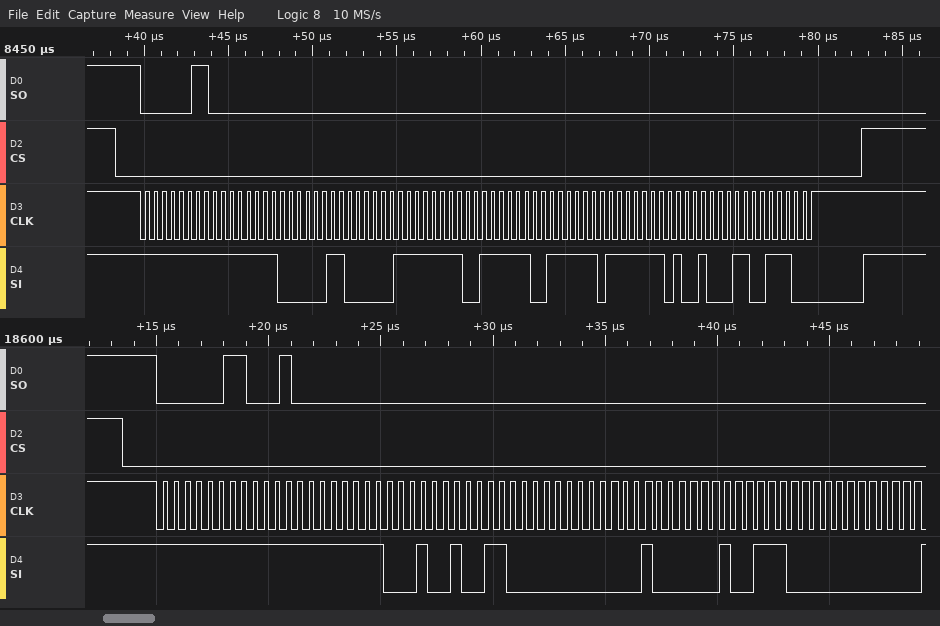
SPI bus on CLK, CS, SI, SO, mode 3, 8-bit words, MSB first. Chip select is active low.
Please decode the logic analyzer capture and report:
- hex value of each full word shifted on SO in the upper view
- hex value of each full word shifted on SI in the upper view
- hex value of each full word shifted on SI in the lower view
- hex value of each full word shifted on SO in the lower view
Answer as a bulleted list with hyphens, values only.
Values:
- 03, 00, 00, 00, 00, 00, 00, 00, 00, 00
- FF, FF, 03, 03, FC, FC, FD, FD, 23, 38
- FF, FF, F1, 26, 00, 10, 27, 00
- 03, 10, 00, 00, 00, 00, 00, 00
